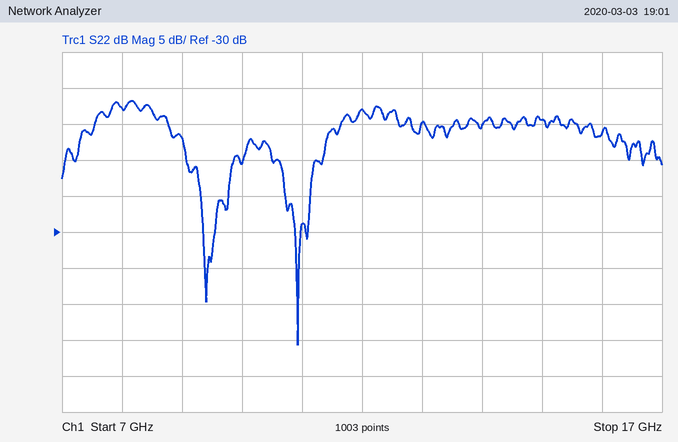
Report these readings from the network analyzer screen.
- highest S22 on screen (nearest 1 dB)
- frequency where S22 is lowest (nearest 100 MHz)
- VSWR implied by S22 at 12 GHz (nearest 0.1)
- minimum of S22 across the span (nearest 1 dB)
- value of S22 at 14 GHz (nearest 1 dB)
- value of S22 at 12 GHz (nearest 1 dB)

-12 dB
10.9 GHz
1.6
-46 dB
-15 dB
-13 dB
